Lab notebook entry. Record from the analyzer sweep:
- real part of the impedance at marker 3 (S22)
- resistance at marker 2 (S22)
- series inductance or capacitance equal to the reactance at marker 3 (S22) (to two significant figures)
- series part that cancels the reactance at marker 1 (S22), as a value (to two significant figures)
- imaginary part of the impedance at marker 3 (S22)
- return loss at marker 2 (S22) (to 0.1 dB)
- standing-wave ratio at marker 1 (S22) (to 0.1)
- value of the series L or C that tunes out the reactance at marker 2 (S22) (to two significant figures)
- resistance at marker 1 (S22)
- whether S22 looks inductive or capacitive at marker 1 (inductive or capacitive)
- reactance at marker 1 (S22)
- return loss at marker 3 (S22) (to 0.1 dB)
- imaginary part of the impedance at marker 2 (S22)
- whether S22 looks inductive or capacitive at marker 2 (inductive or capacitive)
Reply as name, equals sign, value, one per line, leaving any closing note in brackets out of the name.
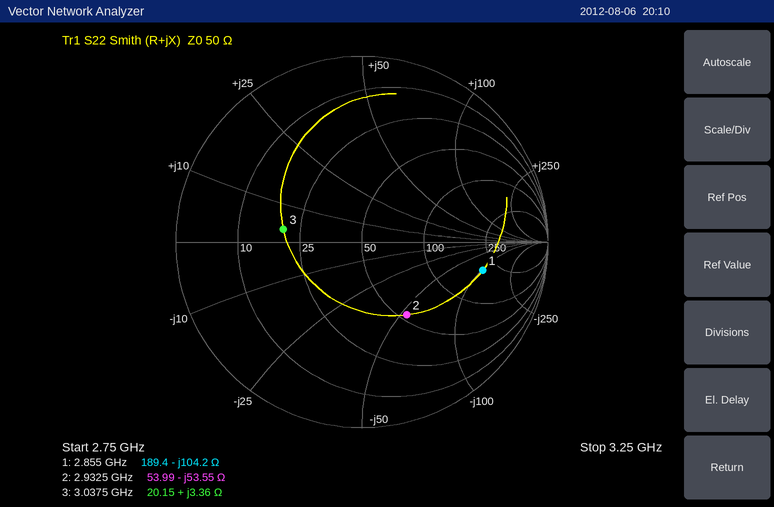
real part of the impedance at marker 3 = 20.15 Ω
resistance at marker 2 = 53.99 Ω
series inductance or capacitance equal to the reactance at marker 3 (S22) = 180 pH
series part that cancels the reactance at marker 1 (S22), as a value = 5.8 nH
imaginary part of the impedance at marker 3 = +3.36 Ω
return loss at marker 2 (S22) = 6.8 dB
standing-wave ratio at marker 1 (S22) = 5.0
value of the series L or C that tunes out the reactance at marker 2 (S22) = 2.9 nH
resistance at marker 1 = 189.4 Ω
whether S22 looks inductive or capacitive at marker 1 = capacitive
reactance at marker 1 = -104.2 Ω
return loss at marker 3 (S22) = 7.4 dB
imaginary part of the impedance at marker 2 = -53.55 Ω
whether S22 looks inductive or capacitive at marker 2 = capacitive
